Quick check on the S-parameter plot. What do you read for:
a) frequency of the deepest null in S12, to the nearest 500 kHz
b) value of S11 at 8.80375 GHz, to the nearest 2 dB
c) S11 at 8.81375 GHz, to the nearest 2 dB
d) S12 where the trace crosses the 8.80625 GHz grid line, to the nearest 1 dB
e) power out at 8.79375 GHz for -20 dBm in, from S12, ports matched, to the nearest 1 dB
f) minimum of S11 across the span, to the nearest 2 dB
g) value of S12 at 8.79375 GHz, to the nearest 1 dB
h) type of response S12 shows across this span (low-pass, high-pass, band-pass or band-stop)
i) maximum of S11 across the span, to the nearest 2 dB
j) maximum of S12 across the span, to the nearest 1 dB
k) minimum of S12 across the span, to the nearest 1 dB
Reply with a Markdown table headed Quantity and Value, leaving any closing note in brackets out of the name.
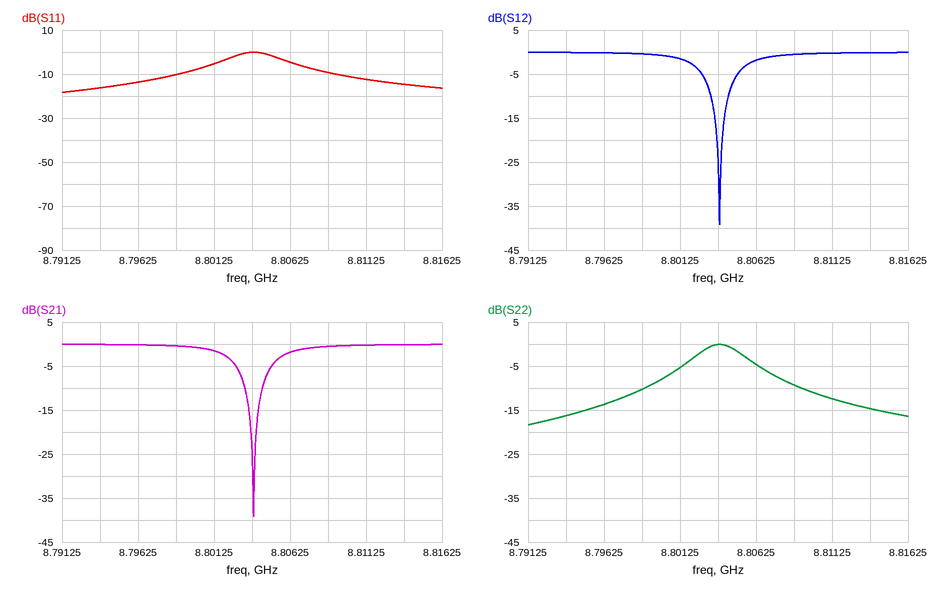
| Quantity | Value |
|---|---|
| frequency of the deepest null in S12, to the nearest 500 kHz | 8.8040 GHz |
| value of S11 at 8.80375 GHz, to the nearest 2 dB | 0 dB |
| S11 at 8.81375 GHz, to the nearest 2 dB | -14 dB |
| S12 where the trace crosses the 8.80625 GHz grid line, to the nearest 1 dB | -2 dB |
| power out at 8.79375 GHz for -20 dBm in, from S12, ports matched, to the nearest 1 dB | -20 dBm |
| minimum of S11 across the span, to the nearest 2 dB | -18 dB |
| value of S12 at 8.79375 GHz, to the nearest 1 dB | 0 dB |
| type of response S12 shows across this span | band-stop |
| maximum of S11 across the span, to the nearest 2 dB | 0 dB |
| maximum of S12 across the span, to the nearest 1 dB | 0 dB |
| minimum of S12 across the span, to the nearest 1 dB | -39 dB |
